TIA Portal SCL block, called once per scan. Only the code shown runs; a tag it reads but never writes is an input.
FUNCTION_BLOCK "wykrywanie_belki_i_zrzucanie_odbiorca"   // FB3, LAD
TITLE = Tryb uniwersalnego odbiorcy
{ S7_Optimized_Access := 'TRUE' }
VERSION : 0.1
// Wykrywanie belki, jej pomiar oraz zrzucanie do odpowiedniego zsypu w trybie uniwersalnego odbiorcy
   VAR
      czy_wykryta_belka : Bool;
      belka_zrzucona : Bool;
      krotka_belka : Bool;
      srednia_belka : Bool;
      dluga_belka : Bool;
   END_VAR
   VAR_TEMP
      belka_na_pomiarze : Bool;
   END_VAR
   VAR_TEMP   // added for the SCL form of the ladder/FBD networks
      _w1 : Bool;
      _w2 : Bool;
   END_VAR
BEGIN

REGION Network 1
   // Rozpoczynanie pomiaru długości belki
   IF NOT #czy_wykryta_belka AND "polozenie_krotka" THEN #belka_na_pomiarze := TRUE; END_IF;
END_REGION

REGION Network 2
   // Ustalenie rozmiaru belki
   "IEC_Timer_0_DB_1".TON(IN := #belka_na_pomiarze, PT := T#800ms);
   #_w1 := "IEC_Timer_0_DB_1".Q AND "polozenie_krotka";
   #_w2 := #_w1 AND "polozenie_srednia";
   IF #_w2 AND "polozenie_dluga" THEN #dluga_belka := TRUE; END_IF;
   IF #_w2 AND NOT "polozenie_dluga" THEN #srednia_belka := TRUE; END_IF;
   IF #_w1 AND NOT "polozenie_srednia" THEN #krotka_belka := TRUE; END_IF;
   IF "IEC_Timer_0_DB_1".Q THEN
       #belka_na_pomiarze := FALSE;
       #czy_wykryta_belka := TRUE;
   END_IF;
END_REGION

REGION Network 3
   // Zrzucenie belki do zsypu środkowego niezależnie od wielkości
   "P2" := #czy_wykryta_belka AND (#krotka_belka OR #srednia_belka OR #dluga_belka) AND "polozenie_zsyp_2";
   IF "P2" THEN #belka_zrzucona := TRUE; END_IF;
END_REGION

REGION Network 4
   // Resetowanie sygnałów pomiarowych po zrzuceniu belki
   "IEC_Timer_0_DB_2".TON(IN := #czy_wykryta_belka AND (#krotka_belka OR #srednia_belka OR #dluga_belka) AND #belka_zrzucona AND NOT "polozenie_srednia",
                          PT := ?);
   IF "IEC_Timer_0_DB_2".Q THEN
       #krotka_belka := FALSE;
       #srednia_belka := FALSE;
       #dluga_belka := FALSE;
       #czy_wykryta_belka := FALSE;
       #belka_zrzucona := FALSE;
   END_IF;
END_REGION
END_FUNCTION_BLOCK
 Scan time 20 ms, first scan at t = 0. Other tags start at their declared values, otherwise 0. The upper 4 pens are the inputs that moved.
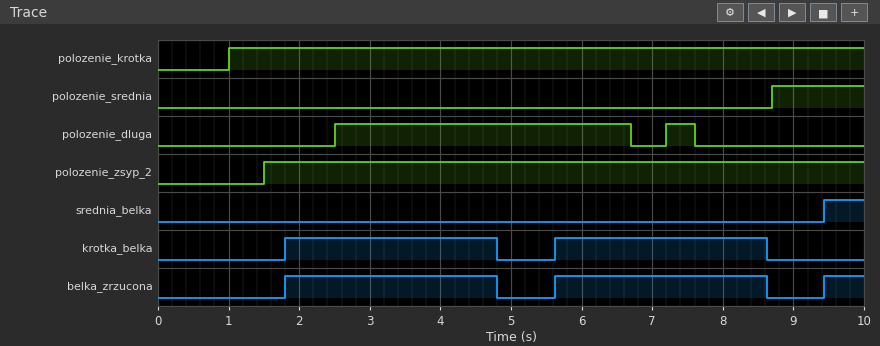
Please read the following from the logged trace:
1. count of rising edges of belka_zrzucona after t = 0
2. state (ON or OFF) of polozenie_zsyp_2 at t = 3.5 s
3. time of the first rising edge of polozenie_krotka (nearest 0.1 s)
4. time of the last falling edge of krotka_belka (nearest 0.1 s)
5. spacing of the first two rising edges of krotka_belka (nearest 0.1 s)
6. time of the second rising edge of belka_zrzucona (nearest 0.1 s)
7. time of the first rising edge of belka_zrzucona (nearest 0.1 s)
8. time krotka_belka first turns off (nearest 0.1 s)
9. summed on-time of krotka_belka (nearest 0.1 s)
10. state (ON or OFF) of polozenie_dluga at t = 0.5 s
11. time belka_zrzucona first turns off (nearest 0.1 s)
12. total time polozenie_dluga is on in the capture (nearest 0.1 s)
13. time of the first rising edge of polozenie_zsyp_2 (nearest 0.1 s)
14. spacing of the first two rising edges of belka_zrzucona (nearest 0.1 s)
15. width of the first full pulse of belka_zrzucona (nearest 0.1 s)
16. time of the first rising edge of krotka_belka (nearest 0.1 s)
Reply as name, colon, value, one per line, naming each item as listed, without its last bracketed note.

count of rising edges of belka_zrzucona after t = 0: 3
state (ON or OFF) of polozenie_zsyp_2 at t = 3.5 s: ON
time of the first rising edge of polozenie_krotka: 1.0 s
time of the last falling edge of krotka_belka: 8.6 s
spacing of the first two rising edges of krotka_belka: 3.8 s
time of the second rising edge of belka_zrzucona: 5.6 s
time of the first rising edge of belka_zrzucona: 1.8 s
time krotka_belka first turns off: 4.8 s
summed on-time of krotka_belka: 6.0 s
state (ON or OFF) of polozenie_dluga at t = 0.5 s: OFF
time belka_zrzucona first turns off: 4.8 s
total time polozenie_dluga is on in the capture: 4.6 s
time of the first rising edge of polozenie_zsyp_2: 1.5 s
spacing of the first two rising edges of belka_zrzucona: 3.8 s
width of the first full pulse of belka_zrzucona: 3.0 s
time of the first rising edge of krotka_belka: 1.8 s
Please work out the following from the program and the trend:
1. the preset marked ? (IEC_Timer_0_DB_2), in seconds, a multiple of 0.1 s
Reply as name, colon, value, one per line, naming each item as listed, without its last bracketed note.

the preset marked ? (IEC_Timer_0_DB_2), in seconds, a multiple of 0.1 s: 3.0 s
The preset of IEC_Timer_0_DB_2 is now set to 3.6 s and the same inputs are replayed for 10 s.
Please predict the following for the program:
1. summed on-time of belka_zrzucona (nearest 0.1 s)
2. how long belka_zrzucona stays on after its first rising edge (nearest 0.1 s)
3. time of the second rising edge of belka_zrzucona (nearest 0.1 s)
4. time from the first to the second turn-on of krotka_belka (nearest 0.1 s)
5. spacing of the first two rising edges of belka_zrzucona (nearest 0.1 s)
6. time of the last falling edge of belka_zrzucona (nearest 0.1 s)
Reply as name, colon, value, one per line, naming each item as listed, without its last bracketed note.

summed on-time of belka_zrzucona: 7.4 s
how long belka_zrzucona stays on after its first rising edge: 3.6 s
time of the second rising edge of belka_zrzucona: 6.2 s
time from the first to the second turn-on of krotka_belka: 4.4 s
spacing of the first two rising edges of belka_zrzucona: 4.4 s
time of the last falling edge of belka_zrzucona: 5.4 s
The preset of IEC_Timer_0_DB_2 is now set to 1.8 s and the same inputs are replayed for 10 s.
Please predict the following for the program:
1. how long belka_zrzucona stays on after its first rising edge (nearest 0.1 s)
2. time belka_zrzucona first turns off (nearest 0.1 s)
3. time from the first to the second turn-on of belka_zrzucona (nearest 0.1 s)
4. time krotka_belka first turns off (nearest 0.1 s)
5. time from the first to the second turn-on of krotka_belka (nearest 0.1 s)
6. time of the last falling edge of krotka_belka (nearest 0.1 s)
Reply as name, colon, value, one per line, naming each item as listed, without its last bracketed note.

how long belka_zrzucona stays on after its first rising edge: 1.8 s
time belka_zrzucona first turns off: 3.6 s
time from the first to the second turn-on of belka_zrzucona: 2.6 s
time krotka_belka first turns off: 3.6 s
time from the first to the second turn-on of krotka_belka: 2.6 s
time of the last falling edge of krotka_belka: 6.2 s
